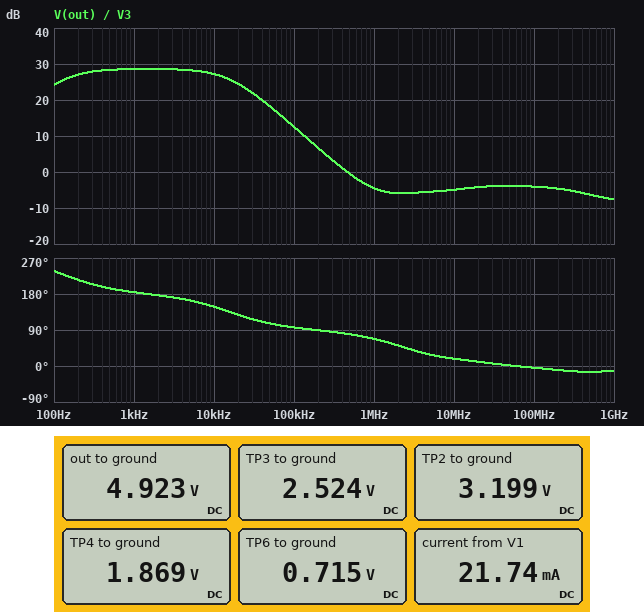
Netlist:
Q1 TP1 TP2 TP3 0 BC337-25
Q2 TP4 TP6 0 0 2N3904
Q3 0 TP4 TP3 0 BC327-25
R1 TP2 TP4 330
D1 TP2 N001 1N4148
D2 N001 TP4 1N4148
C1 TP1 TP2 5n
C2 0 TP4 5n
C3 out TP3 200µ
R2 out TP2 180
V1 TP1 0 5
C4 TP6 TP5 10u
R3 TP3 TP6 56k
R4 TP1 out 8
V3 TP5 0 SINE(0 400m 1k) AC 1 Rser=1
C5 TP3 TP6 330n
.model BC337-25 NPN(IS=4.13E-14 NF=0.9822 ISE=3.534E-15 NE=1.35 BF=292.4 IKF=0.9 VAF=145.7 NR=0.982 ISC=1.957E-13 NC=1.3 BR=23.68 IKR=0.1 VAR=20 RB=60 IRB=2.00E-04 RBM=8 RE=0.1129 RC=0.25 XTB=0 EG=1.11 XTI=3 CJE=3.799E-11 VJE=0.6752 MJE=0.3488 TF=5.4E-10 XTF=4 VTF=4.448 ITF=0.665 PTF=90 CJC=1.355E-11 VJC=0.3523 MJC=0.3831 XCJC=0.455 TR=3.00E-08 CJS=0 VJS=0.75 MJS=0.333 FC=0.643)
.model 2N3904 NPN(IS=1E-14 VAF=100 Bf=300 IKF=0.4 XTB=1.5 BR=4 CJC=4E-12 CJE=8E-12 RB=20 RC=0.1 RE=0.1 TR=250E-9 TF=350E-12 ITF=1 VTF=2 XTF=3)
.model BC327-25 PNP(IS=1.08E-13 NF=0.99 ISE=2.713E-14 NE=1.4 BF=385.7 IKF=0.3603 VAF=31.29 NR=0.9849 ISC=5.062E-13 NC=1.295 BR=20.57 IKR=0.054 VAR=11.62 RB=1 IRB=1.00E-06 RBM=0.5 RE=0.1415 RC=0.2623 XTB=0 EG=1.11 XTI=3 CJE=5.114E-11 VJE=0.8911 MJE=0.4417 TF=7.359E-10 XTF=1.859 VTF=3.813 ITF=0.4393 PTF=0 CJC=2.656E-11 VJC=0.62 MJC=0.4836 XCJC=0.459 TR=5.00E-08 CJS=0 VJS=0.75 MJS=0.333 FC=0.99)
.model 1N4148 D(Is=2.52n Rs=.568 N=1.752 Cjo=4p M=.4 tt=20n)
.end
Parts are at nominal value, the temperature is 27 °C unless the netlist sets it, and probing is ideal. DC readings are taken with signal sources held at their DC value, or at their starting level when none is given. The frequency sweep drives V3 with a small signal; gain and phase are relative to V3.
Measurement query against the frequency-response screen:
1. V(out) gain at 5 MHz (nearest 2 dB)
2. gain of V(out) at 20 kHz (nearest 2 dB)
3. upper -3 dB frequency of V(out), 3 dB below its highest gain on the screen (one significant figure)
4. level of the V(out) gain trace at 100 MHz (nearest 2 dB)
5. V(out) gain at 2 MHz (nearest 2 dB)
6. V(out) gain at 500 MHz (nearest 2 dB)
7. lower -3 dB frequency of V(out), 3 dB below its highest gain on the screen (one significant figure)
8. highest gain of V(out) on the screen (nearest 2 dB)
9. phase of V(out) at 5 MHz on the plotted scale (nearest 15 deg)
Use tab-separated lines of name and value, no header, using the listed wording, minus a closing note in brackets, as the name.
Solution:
V(out) gain at 5 MHz	-6 dB
gain of V(out) at 20 kHz	24 dB
upper -3 dB frequency of V(out), 3 dB below its highest gain on the screen	20 kHz
level of the V(out) gain trace at 100 MHz	-4 dB
V(out) gain at 2 MHz	-6 dB
V(out) gain at 500 MHz	-6 dB
lower -3 dB frequency of V(out), 3 dB below its highest gain on the screen	100 Hz
highest gain of V(out) on the screen	28 dB
phase of V(out) at 5 MHz on the plotted scale	30 deg
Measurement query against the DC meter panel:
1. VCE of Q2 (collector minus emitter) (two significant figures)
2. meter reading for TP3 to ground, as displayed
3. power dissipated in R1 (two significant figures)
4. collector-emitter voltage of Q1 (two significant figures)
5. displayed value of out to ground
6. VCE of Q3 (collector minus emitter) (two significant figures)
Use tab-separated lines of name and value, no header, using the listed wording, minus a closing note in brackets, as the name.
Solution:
VCE of Q2 (collector minus emitter)	1.9 V
meter reading for TP3 to ground, as displayed	2.524 V
power dissipated in R1	5.4 mW
collector-emitter voltage of Q1	2.5 V
displayed value of out to ground	4.923 V
VCE of Q3 (collector minus emitter)	-2.5 V
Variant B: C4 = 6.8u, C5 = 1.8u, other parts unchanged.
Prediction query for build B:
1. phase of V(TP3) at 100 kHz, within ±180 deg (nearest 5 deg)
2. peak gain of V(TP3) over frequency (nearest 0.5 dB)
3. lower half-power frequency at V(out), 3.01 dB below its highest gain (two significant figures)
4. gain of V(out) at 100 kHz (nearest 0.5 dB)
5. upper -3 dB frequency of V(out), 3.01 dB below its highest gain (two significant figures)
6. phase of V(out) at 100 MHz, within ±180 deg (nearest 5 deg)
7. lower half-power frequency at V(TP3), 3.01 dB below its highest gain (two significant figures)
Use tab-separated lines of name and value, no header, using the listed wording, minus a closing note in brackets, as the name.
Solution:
phase of V(TP3) at 100 kHz, within ±180 deg	100 deg
peak gain of V(TP3) over frequency	11.5 dB
lower half-power frequency at V(out), 3.01 dB below its highest gain	110 Hz
gain of V(out) at 100 kHz	-1.5 dB
upper -3 dB frequency of V(out), 3.01 dB below its highest gain	23 kHz
phase of V(out) at 100 MHz, within ±180 deg	-5 deg
lower half-power frequency at V(TP3), 3.01 dB below its highest gain	3.3 Hz
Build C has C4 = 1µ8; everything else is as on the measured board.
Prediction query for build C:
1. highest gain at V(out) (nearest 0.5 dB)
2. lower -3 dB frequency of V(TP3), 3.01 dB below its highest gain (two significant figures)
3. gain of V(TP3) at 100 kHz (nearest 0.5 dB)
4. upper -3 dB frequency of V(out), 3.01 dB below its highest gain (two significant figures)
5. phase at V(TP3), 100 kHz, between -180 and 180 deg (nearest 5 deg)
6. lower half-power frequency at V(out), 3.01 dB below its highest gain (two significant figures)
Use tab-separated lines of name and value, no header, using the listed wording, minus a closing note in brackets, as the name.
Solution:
highest gain at V(out)	14.5 dB
lower -3 dB frequency of V(TP3), 3.01 dB below its highest gain	17 Hz
gain of V(TP3) at 100 kHz	10.5 dB
upper -3 dB frequency of V(out), 3.01 dB below its highest gain	82 kHz
phase at V(TP3), 100 kHz, between -180 and 180 deg	125 deg
lower half-power frequency at V(out), 3.01 dB below its highest gain	110 Hz
